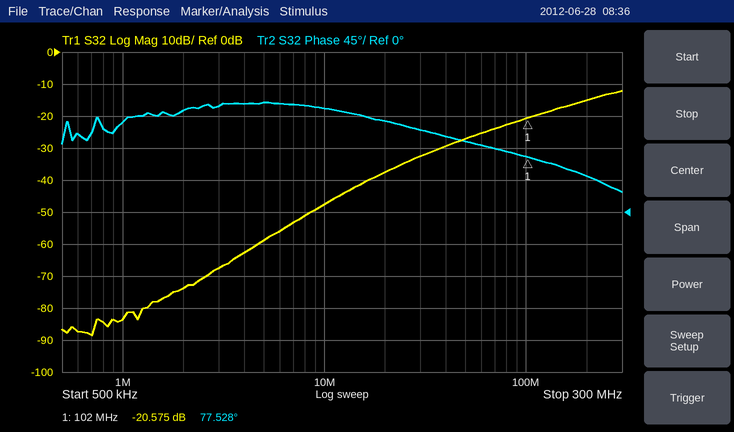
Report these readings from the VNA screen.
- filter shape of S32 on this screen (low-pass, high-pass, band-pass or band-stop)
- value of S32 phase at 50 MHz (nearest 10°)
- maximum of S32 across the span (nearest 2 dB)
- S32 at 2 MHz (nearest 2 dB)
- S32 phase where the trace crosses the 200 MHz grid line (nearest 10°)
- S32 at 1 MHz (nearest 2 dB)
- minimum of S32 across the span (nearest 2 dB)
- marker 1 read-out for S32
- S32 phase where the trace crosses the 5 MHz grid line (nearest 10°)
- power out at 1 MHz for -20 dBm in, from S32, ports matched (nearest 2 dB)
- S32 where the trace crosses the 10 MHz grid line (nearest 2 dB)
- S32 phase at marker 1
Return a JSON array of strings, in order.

["high-pass", "100°", "-12 dB", "-74 dB", "50°", "-84 dB", "-88 dB", "-20.575 dB", "150°", "-104 dBm", "-48 dB", "77.528°"]
